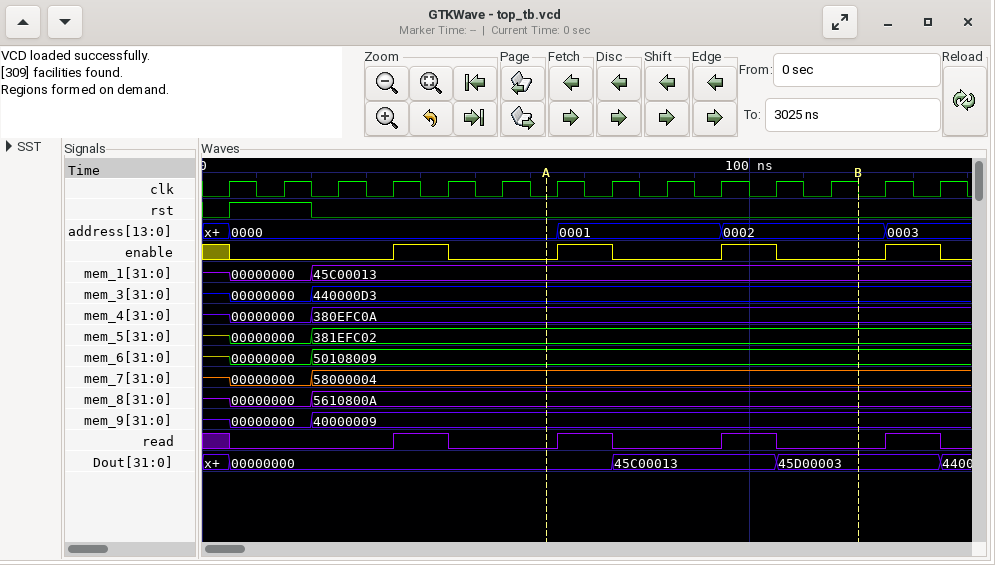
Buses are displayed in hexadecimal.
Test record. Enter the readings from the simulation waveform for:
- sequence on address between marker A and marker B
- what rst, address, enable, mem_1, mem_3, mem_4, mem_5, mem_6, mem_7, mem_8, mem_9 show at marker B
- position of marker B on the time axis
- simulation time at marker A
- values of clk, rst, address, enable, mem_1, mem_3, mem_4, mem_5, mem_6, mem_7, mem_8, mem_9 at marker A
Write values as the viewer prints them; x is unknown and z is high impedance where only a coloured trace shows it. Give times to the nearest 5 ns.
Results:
0000, 0001, 0002
rst=0, address=0002, enable=0, mem_1=45C00013, mem_3=440000D3, mem_4=380EFC0A, mem_5=381EFC02, mem_6=50108009, mem_7=58000004, mem_8=5610800A, mem_9=40000009
120 ns
65 ns
clk=0, rst=0, address=0000, enable=0, mem_1=45C00013, mem_3=440000D3, mem_4=380EFC0A, mem_5=381EFC02, mem_6=50108009, mem_7=58000004, mem_8=5610800A, mem_9=40000009
